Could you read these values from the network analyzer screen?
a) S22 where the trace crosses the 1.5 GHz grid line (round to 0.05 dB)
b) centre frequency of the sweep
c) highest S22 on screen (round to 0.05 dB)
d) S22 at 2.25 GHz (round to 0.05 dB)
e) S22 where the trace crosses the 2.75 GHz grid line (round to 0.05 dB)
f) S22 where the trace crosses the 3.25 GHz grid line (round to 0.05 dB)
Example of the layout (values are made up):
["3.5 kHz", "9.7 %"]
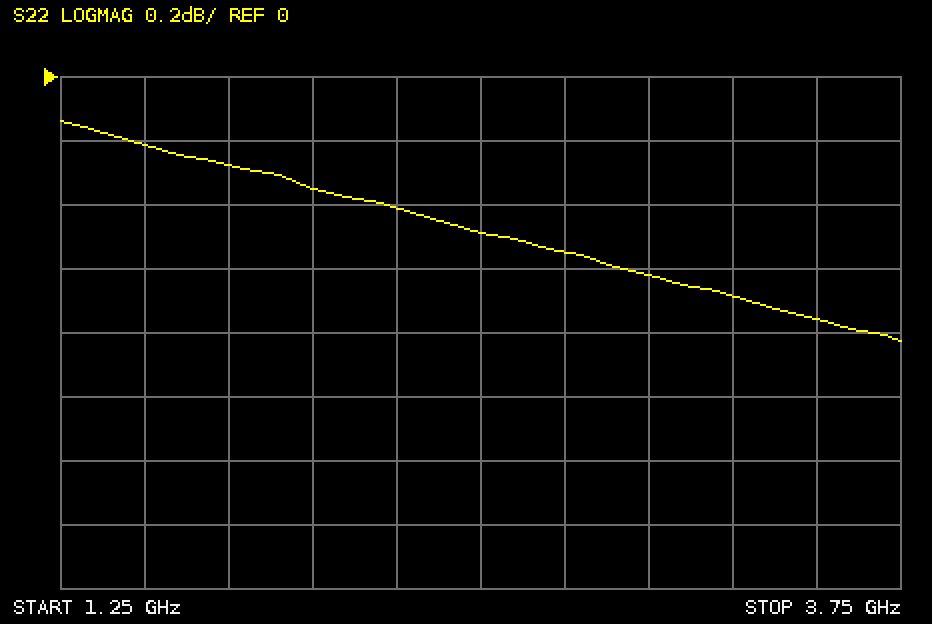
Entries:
["-0.20 dB", "2.5 GHz", "-0.15 dB", "-0.40 dB", "-0.55 dB", "-0.70 dB"]
